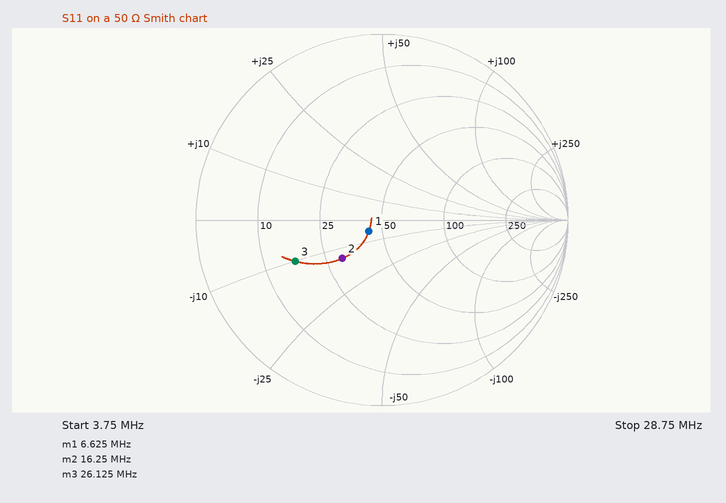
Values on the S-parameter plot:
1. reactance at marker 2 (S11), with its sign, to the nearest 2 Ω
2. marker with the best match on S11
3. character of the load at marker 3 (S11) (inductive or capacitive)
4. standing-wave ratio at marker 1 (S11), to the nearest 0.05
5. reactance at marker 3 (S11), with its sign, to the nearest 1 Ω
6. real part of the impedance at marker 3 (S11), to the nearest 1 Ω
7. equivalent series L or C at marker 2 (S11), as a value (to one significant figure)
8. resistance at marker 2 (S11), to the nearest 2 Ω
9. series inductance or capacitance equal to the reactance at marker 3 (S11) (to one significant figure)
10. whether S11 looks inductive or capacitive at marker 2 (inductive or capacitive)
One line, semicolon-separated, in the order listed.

-14 Ω; marker 1; capacitive; 1.20; -10 Ω; 17 Ω; 700 pF; 30 Ω; 600 pF; capacitive
